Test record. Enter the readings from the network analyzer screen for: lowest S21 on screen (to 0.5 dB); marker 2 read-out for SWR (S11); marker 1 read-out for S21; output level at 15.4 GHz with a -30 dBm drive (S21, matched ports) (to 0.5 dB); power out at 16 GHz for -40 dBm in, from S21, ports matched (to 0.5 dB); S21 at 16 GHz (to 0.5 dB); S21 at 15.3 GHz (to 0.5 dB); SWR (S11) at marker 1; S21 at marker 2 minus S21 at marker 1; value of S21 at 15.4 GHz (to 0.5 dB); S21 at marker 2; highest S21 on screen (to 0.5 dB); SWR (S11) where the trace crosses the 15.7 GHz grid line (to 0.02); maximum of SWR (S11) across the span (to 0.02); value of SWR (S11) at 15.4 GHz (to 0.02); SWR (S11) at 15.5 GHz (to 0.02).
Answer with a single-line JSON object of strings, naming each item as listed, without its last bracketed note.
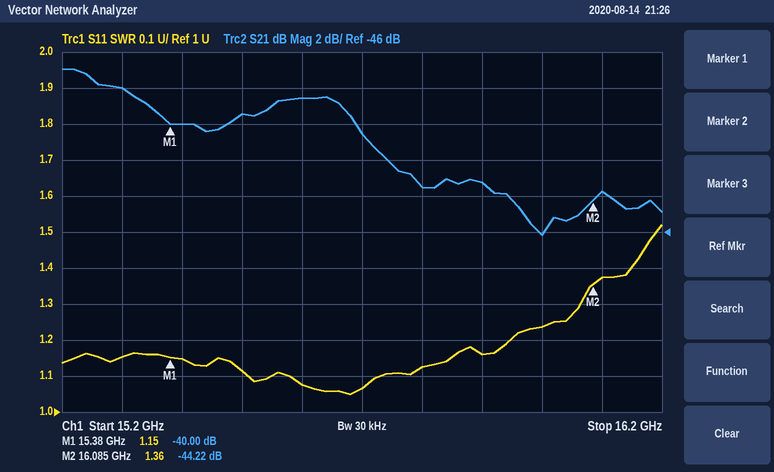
{"lowest S21 on screen": "-46.0 dB", "marker 2 read-out for SWR": "1.36", "marker 1 read-out for S21": "-40.00 dB", "output level at 15.4 GHz with a -30 dBm drive (S21, matched ports)": "-70.0 dBm", "power out at 16 GHz for -40 dBm in, from S21, ports matched": "-86.0 dBm", "S21 at 16 GHz": "-46.0 dB", "S21 at 15.3 GHz": "-38.0 dB", "SWR (S11) at marker 1": "1.15", "S21 at marker 2 minus S21 at marker 1": "-4.22 dB", "value of S21 at 15.4 GHz": "-40.0 dB", "S21 at marker 2": "-44.22 dB", "highest S21 on screen": "-37.0 dB", "SWR (S11) where the trace crosses the 15.7 GHz grid line": "1.06", "maximum of SWR (S11) across the span": "1.52", "value of SWR (S11) at 15.4 GHz": "1.14", "SWR (S11) at 15.5 GHz": "1.12"}
